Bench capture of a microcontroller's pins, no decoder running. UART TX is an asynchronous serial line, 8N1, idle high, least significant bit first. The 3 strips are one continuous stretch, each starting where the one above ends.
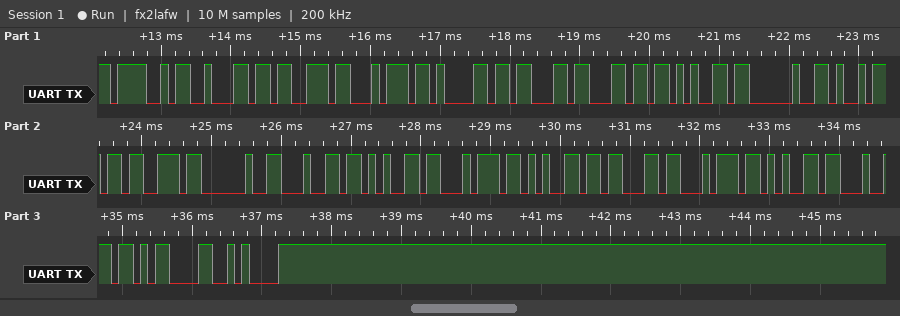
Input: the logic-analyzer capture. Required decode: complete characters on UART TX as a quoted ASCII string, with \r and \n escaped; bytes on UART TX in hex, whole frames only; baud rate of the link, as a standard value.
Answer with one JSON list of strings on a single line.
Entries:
["\"Obstacle is detected\\r\\n\"", "4F 62 73 74 61 63 6C 65 20 69 73 20 64 65 74 65 63 74 65 64 0D 0A", "9600 baud"]
